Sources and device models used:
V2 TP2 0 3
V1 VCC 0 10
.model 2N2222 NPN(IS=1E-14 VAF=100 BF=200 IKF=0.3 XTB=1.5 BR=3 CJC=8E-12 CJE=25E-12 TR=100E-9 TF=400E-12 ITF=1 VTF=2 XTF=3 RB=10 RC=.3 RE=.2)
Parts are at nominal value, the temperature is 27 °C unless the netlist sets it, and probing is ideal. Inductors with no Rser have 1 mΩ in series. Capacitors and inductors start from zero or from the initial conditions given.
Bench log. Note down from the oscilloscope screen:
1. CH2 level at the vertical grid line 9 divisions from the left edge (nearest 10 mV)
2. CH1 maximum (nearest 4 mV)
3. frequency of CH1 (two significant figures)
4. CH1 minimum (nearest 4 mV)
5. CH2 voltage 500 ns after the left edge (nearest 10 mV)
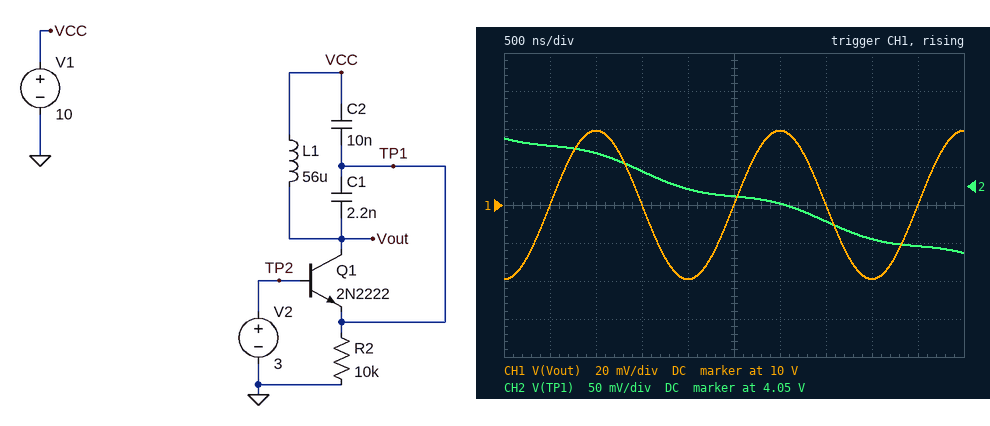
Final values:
3.97 V
10.040 V
500 kHz
9.960 V
4.10 V
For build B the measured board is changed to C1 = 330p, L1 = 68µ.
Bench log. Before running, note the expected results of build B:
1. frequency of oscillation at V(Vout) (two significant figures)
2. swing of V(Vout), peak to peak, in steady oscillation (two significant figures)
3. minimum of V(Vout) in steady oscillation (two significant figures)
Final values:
1.1 MHz
230 mV
9.9 V
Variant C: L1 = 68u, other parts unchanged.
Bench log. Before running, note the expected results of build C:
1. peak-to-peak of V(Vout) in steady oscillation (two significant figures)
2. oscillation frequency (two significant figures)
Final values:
83 mV
450 kHz
